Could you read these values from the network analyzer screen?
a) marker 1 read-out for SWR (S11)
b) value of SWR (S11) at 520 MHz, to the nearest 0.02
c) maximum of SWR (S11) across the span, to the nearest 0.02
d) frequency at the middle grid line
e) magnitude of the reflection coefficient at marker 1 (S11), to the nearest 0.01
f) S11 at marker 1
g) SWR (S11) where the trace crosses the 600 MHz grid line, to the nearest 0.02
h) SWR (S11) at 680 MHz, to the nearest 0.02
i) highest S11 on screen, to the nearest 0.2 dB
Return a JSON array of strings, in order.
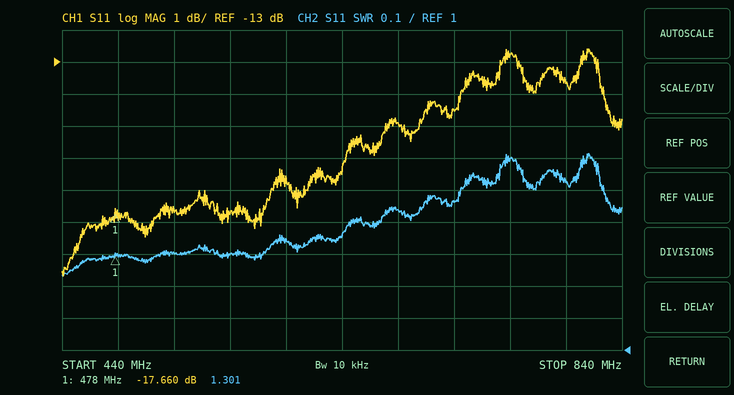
["1.301", "1.30", "1.62", "640 MHz", "0.13", "-17.660 dB", "1.34", "1.44", "-12.6 dB"]
